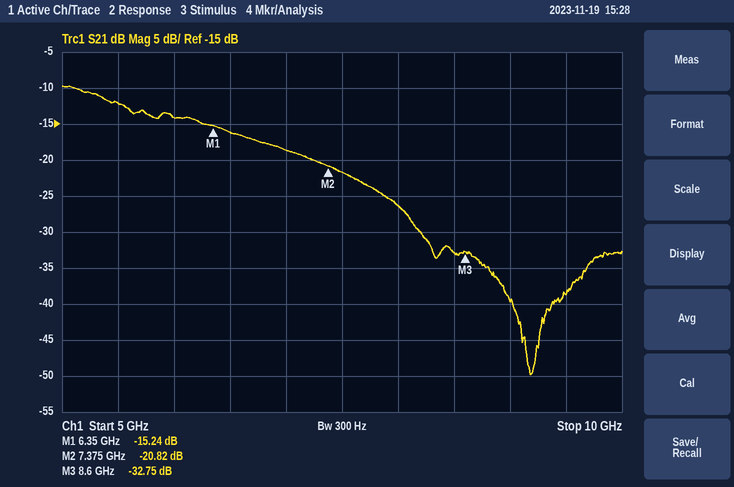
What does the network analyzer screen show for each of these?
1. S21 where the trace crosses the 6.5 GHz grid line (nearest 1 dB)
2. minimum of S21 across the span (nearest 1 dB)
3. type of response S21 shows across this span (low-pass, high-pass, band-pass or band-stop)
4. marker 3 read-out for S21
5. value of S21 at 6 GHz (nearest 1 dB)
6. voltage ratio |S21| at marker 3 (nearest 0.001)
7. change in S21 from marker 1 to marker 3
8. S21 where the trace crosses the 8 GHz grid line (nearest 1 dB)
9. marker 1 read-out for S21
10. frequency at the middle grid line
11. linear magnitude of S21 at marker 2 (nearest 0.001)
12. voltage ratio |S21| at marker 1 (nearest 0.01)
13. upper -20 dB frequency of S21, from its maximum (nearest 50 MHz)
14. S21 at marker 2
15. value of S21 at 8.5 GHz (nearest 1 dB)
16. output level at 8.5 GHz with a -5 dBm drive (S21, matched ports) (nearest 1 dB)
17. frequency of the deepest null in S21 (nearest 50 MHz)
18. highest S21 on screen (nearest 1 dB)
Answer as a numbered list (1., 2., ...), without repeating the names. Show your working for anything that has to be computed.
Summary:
1. -16 dB
2. -50 dB
3. low-pass
4. -32.75 dB
5. -14 dB
6. 10^(-32.75/20) ≈ 0.023
7. -32.75 − (-15.24) = -17.51 dB
8. -26 dB
9. -15.24 dB
10. 7.5 GHz
11. 10^(-20.82/20) ≈ 0.091
12. 10^(-15.24/20) ≈ 0.17
13. 8.20 GHz
14. -20.82 dB
15. -33 dB
16. -5 dBm + (-33 dB) = -38 dBm
17. 9.20 GHz
18. -10 dB
